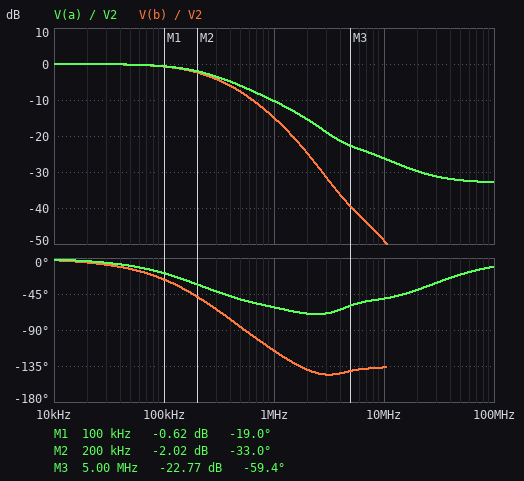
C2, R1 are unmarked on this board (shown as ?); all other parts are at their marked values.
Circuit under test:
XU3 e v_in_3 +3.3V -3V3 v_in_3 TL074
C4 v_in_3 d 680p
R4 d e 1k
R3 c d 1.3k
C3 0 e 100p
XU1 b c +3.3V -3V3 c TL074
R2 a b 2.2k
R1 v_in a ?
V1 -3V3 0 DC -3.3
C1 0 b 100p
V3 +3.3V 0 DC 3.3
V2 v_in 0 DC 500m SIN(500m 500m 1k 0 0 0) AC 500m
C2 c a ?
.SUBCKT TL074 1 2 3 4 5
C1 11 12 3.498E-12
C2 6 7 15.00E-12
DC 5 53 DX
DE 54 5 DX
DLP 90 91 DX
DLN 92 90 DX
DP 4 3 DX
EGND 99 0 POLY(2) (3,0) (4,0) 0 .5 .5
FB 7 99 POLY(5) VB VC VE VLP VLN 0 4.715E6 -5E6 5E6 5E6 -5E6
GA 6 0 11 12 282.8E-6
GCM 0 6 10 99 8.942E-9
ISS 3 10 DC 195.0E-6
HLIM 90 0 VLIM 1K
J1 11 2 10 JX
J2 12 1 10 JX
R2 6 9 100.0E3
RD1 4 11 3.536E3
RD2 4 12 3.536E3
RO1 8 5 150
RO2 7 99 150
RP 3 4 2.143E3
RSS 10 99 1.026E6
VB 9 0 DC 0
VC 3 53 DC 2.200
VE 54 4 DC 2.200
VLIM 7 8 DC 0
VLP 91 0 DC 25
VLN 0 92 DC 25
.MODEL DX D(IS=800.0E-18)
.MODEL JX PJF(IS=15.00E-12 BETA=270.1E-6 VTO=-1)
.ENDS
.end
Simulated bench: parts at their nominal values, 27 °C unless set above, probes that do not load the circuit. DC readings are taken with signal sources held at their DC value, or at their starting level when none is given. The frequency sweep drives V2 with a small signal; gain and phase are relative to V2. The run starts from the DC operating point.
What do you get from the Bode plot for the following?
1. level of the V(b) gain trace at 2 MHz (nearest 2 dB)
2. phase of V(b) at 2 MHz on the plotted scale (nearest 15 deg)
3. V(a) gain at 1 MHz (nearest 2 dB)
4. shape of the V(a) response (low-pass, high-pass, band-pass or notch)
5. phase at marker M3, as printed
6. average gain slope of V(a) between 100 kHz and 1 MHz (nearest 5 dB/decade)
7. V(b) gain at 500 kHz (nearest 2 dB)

-24 dB
-135 deg
-10 dB
low-pass
-59.4 deg
-10 dB/decade
-8 dB
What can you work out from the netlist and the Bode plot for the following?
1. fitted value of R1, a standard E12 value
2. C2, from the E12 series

5.6 kΩ
56 pF
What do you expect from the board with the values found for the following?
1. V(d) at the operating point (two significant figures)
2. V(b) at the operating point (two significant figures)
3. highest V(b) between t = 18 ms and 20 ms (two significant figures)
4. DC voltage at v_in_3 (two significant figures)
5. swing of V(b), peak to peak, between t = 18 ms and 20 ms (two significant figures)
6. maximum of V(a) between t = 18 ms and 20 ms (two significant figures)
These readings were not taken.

500 mV
500 mV
1.0 V
500 mV
1.0 V
1.0 V
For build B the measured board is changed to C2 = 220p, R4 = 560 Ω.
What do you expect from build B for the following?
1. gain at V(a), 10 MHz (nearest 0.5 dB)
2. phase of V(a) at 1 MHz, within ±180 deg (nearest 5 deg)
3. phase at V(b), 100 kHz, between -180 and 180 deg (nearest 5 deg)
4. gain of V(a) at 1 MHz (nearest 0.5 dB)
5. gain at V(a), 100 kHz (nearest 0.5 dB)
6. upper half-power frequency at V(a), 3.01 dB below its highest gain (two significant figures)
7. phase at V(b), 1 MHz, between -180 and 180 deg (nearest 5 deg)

-31.5 dB
-105 deg
-30 deg
-18.5 dB
0 dB
310 kHz
-155 deg
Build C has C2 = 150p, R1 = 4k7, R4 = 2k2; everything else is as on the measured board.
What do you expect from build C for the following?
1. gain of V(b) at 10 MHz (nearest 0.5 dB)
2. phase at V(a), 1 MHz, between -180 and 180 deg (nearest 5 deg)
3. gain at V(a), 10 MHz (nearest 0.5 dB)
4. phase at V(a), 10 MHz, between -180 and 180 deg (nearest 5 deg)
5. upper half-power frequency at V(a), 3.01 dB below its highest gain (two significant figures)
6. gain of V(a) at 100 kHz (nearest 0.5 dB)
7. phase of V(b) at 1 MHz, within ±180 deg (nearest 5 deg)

-52.0 dB
-90 deg
-29.5 dB
-25 deg
370 kHz
0 dB
-145 deg
